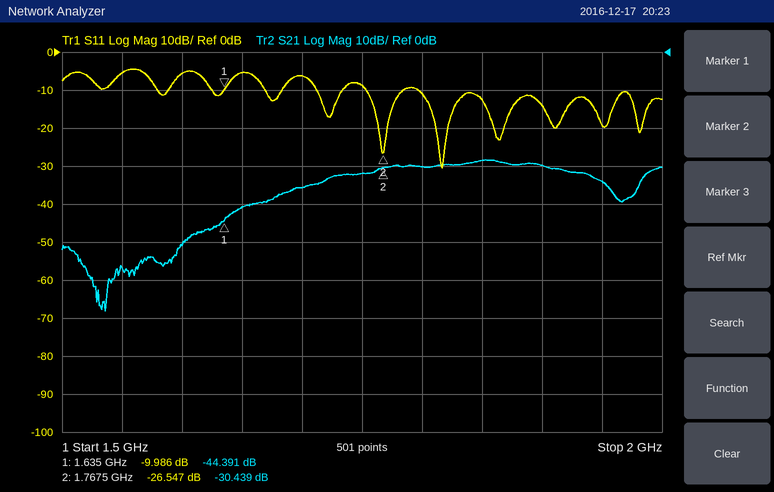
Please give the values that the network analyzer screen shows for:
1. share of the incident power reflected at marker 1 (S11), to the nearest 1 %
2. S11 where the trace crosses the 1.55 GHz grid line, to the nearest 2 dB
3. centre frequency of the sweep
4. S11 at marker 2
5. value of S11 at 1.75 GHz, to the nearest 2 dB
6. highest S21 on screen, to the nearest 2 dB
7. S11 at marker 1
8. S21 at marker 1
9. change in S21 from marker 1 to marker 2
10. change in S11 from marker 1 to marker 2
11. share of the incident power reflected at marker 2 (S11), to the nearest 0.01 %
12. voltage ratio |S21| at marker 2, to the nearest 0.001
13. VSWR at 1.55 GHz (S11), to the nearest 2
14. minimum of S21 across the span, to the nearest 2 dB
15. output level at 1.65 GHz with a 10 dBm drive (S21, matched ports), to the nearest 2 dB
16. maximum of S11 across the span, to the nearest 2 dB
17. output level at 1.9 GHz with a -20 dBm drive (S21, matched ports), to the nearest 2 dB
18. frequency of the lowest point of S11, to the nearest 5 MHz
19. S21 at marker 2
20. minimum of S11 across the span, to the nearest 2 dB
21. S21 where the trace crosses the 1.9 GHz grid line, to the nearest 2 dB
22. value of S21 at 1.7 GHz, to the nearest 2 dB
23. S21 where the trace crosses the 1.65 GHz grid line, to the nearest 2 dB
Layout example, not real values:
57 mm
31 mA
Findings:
10 %
-6 dB
1.75 GHz
-26.547 dB
-8 dB
-28 dB
-9.986 dB
-44.391 dB
13.952 dB
-16.561 dB
0.22 %
0.030
4
-68 dB
-30 dBm
-4 dB
-50 dBm
1.815 GHz
-30.439 dB
-30 dB
-30 dB
-36 dB
-40 dB
